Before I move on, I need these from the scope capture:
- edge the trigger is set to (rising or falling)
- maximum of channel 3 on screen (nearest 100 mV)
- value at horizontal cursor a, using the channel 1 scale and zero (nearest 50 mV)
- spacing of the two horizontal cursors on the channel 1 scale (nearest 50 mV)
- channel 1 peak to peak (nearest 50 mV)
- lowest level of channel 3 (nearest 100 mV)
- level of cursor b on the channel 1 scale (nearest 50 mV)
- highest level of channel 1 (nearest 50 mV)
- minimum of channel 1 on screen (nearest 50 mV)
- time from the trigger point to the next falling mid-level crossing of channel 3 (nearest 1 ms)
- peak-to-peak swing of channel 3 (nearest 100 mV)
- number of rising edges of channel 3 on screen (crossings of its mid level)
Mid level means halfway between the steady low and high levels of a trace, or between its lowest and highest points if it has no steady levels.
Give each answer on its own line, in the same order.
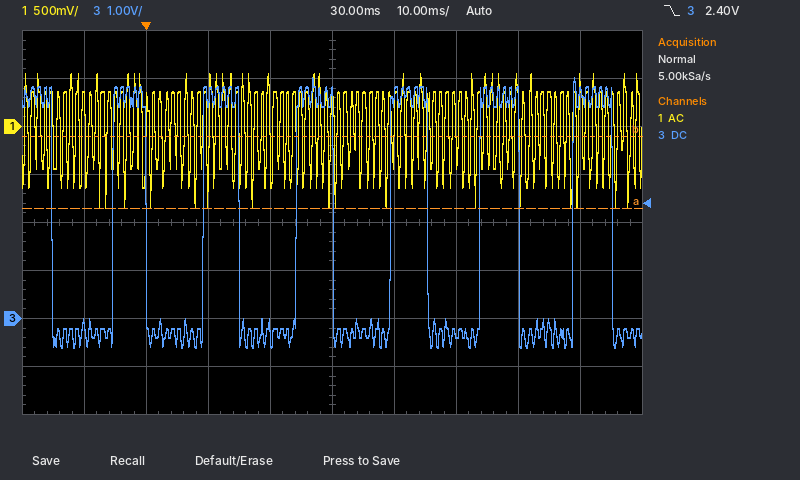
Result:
falling
5.0 V
-850 mV
750 mV
1.40 V
-600 mV
-100 mV
550 mV
-850 mV
15 ms
5.6 V
6
